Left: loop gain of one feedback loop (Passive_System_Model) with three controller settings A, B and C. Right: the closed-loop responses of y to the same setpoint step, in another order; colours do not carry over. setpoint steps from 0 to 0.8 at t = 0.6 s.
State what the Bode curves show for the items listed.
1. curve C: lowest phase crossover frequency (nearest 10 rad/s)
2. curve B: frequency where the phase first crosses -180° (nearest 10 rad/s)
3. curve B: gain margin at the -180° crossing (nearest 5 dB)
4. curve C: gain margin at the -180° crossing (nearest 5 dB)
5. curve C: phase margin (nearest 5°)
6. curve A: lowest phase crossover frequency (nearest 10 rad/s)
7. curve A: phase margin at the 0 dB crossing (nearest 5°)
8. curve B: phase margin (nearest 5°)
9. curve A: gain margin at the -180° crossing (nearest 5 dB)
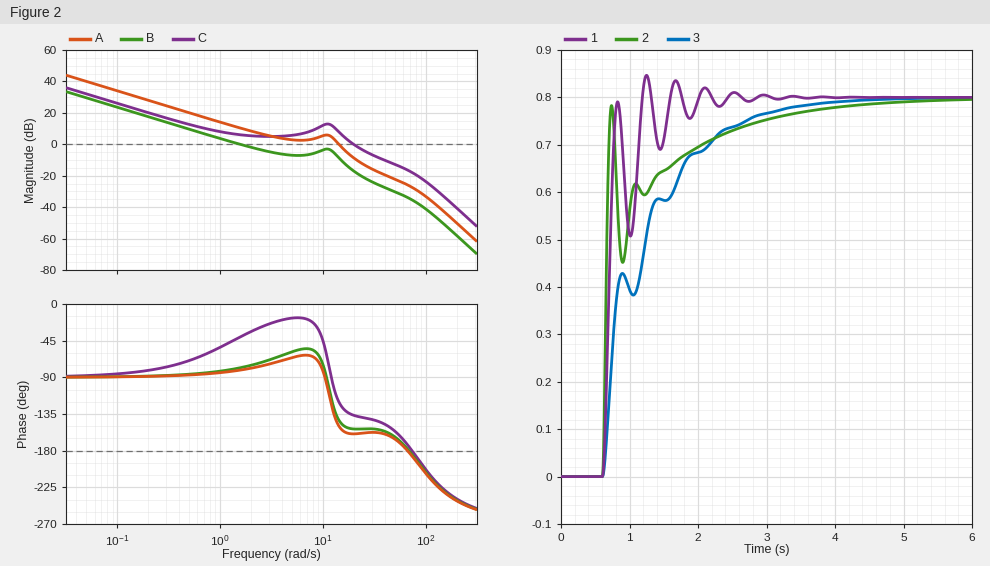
70 rad/s
70 rad/s
35 dB
20 dB
45°
70 rad/s
30°
100°
25 dB
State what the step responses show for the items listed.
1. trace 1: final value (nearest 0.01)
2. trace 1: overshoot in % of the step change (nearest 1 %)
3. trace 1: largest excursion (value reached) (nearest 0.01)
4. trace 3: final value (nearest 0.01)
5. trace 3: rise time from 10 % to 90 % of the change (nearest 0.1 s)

0.80
6 %
0.85
0.80
1.6 s
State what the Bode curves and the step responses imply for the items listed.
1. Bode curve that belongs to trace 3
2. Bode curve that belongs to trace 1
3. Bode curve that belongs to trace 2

B
A
C
